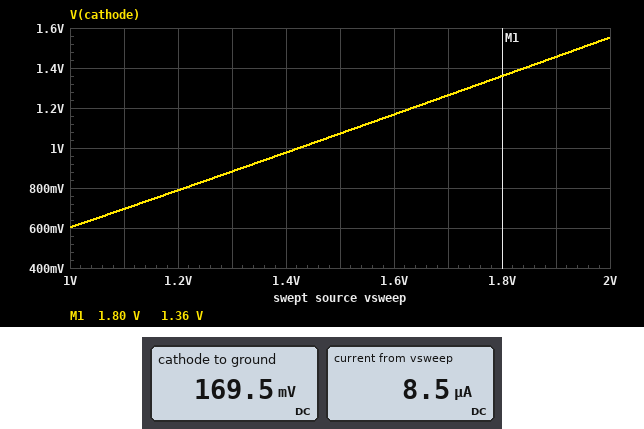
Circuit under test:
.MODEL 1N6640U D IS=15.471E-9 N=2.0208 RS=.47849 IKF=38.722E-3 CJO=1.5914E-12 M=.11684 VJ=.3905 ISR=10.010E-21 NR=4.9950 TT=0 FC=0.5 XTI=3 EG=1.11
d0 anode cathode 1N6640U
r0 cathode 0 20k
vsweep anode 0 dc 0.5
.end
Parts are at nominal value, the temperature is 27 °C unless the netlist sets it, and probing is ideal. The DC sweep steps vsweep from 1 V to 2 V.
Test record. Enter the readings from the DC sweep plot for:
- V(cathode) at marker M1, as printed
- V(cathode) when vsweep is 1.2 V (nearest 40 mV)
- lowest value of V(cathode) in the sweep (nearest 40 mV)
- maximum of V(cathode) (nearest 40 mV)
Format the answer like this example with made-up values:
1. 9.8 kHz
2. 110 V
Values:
1. 1.36 V
2. 800 mV
3. 600 mV
4. 1.56 V
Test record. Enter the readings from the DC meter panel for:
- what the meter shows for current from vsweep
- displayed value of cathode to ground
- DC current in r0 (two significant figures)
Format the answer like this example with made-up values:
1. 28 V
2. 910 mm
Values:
1. 8.5 µA
2. 169.5 mV
3. 8.5 µA
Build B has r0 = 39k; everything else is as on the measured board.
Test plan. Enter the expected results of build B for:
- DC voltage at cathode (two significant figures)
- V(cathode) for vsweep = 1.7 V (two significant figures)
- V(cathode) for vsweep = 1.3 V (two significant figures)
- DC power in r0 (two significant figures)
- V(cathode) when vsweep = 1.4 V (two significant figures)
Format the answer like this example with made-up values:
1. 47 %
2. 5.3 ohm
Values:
1. 200 mV
2. 1.3 V
3. 920 mV
4. 990 nW
5. 1.0 V
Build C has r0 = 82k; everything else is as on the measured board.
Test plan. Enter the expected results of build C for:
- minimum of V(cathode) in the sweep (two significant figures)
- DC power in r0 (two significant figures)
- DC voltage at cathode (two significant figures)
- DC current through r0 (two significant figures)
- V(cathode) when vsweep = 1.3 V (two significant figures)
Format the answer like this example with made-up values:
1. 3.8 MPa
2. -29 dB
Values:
1. 670 mV
2. 630 nW
3. 230 mV
4. 2.8 µA
5. 950 mV
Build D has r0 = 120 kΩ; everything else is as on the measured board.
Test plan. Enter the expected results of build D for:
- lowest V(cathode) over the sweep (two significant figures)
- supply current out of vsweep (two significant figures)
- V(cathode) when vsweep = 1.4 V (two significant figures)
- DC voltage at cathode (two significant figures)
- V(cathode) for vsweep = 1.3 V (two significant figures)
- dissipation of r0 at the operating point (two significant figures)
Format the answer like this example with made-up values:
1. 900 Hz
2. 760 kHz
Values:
1. 690 mV
2. 2.0 µA
3. 1.1 V
4. 240 mV
5. 970 mV
6. 500 nW
